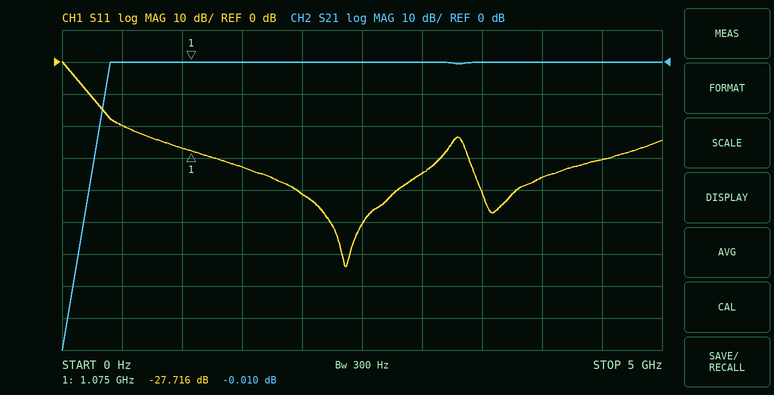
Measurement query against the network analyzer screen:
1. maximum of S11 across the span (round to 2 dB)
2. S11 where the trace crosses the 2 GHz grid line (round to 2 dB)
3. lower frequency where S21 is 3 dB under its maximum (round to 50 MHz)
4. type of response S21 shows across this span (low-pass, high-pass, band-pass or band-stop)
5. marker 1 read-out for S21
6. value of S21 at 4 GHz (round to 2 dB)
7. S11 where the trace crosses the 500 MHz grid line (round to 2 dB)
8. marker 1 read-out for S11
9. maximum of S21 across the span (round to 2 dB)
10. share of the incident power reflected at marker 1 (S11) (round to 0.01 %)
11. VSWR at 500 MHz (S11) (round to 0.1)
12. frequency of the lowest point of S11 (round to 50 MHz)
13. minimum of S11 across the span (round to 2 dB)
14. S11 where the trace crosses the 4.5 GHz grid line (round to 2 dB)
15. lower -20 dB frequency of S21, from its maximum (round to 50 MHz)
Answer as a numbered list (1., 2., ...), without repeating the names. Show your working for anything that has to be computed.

1. 0 dB
2. -42 dB
3. 400 MHz
4. high-pass
5. -0.010 dB
6. 0 dB
7. -20 dB
8. -27.716 dB
9. 0 dB
10. 10^(-27.716/10) ≈ 0.17 %
11. |Γ| = 10^(-20/20) = 0.1000; VSWR = (1 + 0.1000)/(1 − 0.1000) ≈ 1.2
12. 2.35 GHz
13. -64 dB
14. -30 dB
15. 300 MHz
